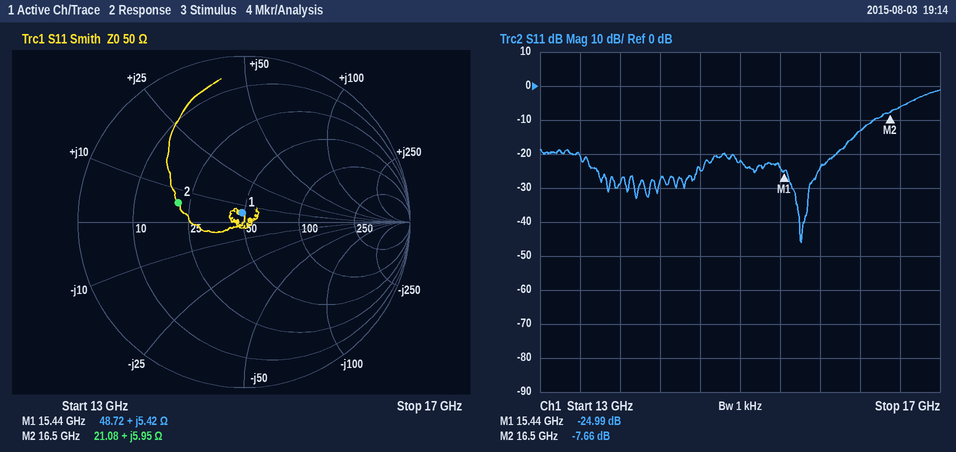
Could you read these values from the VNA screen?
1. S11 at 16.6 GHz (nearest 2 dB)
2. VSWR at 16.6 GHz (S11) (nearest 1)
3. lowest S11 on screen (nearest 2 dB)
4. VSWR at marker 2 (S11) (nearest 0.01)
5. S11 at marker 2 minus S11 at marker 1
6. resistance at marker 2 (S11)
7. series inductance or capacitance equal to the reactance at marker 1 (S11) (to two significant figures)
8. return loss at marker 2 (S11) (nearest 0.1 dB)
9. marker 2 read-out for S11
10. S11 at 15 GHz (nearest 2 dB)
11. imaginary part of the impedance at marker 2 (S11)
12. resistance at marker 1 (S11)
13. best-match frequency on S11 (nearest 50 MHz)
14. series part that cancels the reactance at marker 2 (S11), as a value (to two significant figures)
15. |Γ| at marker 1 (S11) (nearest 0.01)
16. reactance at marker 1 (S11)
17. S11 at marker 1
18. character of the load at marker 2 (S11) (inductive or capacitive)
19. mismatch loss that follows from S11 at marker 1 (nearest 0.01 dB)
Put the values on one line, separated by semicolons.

-6 dB; 3; -46 dB; 2.41; 17.33 dB; 21.08 Ω; 56 pH; 7.7 dB; -7.66 dB; -22 dB; +5.95 Ω; 48.72 Ω; 15.60 GHz; 1.6 pF; 0.06; +5.42 Ω; -24.99 dB; inductive; 0.01 dB
